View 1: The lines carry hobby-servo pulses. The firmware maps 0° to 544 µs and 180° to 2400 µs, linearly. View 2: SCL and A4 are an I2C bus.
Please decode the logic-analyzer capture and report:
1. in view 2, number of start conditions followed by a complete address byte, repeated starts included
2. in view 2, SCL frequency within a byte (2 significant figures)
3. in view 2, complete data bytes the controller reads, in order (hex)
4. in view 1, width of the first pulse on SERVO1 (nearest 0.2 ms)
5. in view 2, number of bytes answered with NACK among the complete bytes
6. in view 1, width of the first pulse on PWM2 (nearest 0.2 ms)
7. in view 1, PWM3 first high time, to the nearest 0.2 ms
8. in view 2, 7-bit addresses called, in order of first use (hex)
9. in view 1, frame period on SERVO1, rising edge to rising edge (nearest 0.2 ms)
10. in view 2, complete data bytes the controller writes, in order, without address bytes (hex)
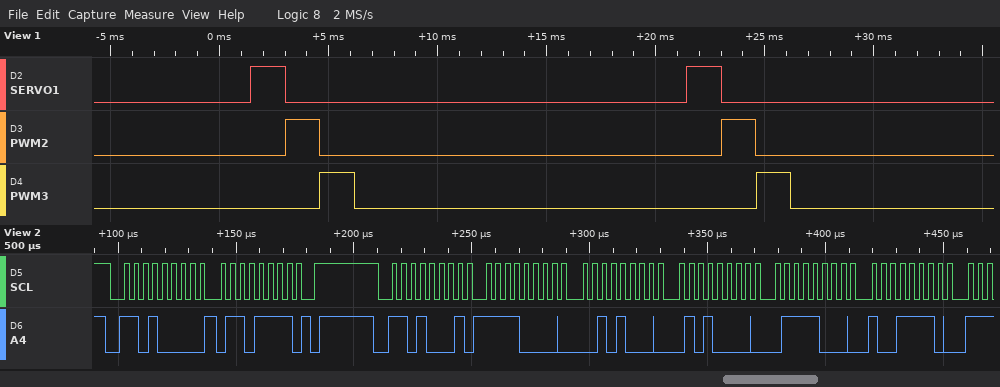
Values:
2
250 kHz
F0 28 50 78 9E
1.6 ms
0
1.6 ms
1.6 ms
0x68
20.0 ms
6F
